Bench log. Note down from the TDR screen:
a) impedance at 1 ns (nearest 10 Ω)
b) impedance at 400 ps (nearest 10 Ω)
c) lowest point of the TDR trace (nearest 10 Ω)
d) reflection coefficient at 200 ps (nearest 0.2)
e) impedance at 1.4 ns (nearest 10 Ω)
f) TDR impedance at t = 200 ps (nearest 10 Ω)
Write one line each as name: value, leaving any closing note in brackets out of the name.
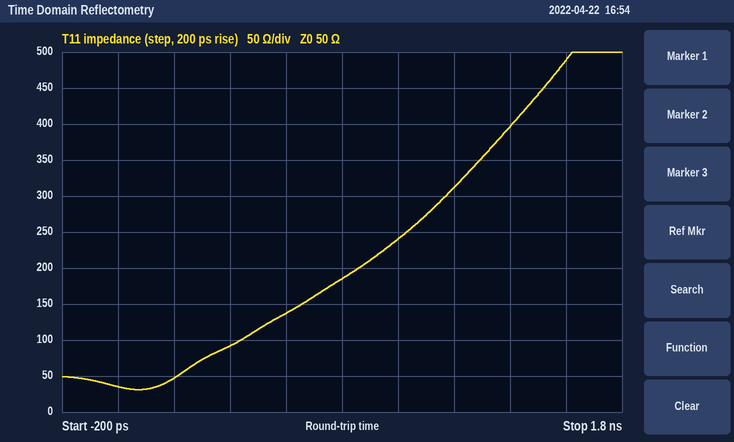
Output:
impedance at 1 ns: 240 Ω
impedance at 400 ps: 90 Ω
lowest point of the TDR trace: 30 Ω
reflection coefficient at 200 ps: 0.0
impedance at 1.4 ns: 400 Ω
TDR impedance at t = 200 ps: 50 Ω
